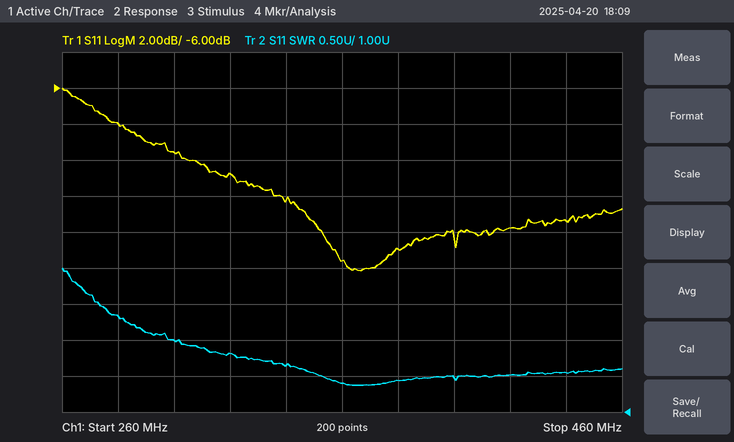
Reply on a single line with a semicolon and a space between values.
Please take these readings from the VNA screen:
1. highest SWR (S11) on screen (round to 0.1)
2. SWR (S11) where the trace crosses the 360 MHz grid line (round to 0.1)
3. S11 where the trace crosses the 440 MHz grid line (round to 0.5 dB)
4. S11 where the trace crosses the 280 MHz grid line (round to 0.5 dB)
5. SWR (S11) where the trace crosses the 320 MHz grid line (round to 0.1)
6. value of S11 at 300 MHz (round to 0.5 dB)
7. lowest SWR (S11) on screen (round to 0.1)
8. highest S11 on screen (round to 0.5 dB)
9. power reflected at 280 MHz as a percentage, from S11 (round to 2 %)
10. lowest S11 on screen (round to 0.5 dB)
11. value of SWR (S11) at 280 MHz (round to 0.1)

3.0; 1.4; -13.5 dB; -8.0 dB; 1.8; -9.5 dB; 1.4; -6.0 dB; 16 %; -16.0 dB; 2.3
